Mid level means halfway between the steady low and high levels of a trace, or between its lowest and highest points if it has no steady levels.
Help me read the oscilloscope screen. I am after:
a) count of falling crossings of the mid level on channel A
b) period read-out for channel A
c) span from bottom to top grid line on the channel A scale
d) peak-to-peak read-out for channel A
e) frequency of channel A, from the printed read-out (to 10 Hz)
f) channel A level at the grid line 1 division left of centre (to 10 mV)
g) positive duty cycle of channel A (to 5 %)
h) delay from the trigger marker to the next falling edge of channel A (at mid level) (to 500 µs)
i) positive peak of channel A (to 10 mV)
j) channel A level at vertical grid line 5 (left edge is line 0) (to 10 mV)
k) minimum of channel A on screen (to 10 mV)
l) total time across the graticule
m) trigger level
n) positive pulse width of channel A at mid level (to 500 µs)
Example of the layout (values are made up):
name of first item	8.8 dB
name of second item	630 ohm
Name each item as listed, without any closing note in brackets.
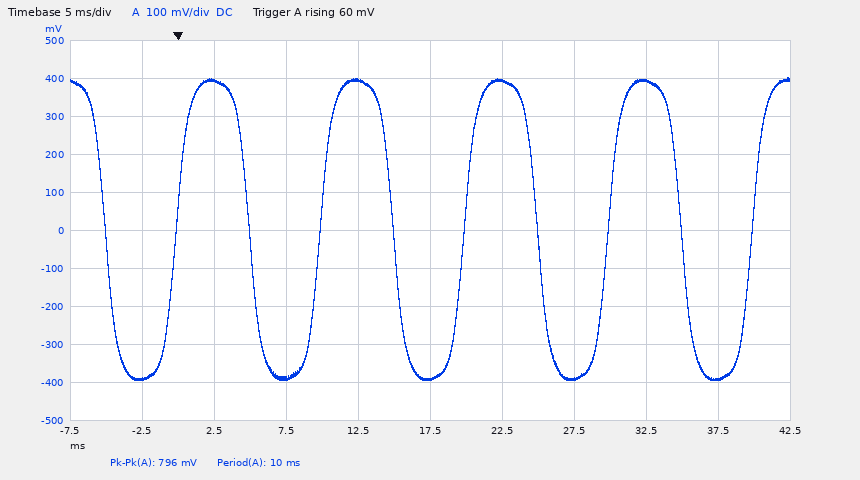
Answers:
count of falling crossings of the mid level on channel A	5
period read-out for channel A	10 ms
span from bottom to top grid line on the channel A scale	1 V
peak-to-peak read-out for channel A	796 mV
frequency of channel A, from the printed read-out	100 Hz
channel A level at the grid line 1 division left of centre	400 mV
positive duty cycle of channel A	50 %
delay from the trigger marker to the next falling edge of channel A (at mid level)	5.0 ms
positive peak of channel A	400 mV
channel A level at vertical grid line 5 (left edge is line 0)	-390 mV
minimum of channel A on screen	-390 mV
total time across the graticule	50 ms
trigger level	60 mV
positive pulse width of channel A at mid level	5.0 ms
